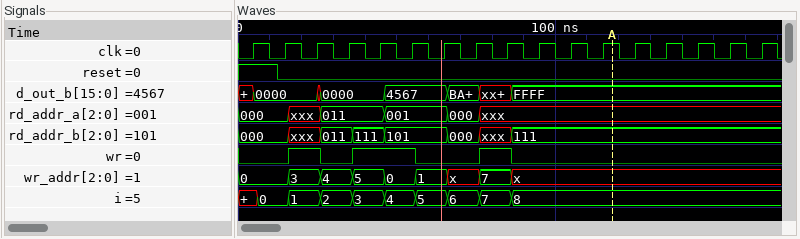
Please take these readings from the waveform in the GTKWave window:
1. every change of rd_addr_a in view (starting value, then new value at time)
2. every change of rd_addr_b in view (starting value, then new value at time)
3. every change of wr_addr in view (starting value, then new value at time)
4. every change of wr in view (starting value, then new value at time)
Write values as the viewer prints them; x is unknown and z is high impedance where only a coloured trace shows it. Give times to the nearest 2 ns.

000, xxx at 16 ns, 011 at 26 ns, 001 at 46 ns, 000 at 66 ns, xxx at 76 ns
000, xxx at 16 ns, 011 at 26 ns, 111 at 36 ns, 101 at 46 ns, 000 at 66 ns, xxx at 76 ns, 111 at 86 ns
0, 3 at 16 ns, 4 at 26 ns, 5 at 36 ns, 0 at 46 ns, 1 at 56 ns, x at 66 ns, 7 at 76 ns, x at 86 ns
0, 1 at 16 ns, 0 at 26 ns, 1 at 36 ns, 0 at 56 ns, 1 at 76 ns, 0 at 86 ns
